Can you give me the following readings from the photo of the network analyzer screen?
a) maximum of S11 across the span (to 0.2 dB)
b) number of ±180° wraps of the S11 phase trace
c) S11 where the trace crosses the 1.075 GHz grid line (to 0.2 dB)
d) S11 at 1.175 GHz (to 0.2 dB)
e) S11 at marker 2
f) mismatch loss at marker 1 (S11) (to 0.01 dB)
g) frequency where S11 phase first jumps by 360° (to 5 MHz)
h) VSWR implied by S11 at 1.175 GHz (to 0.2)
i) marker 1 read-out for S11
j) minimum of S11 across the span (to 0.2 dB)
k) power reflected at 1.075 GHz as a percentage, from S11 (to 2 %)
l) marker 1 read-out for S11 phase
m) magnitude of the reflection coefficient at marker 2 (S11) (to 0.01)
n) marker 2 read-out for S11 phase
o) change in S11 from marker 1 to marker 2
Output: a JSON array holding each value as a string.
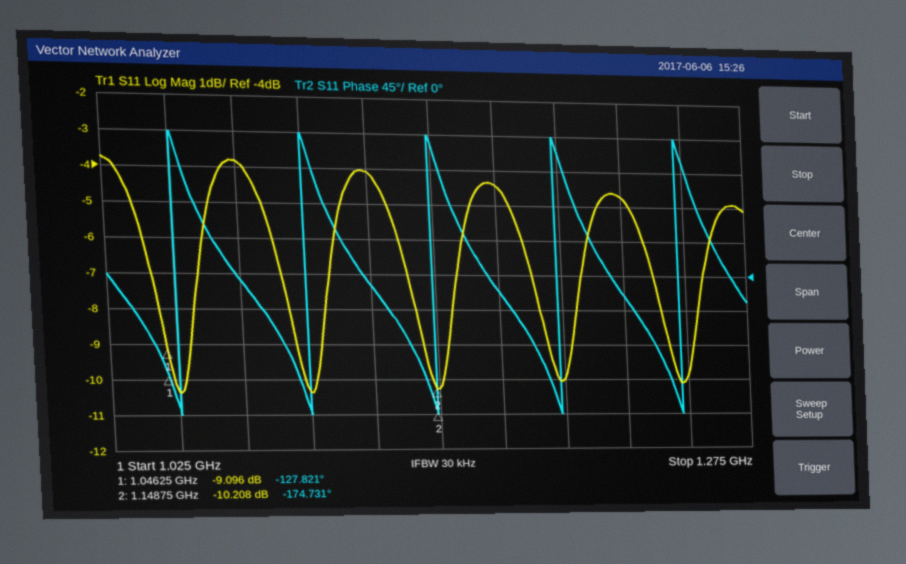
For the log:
["-3.8 dB", "5", "-3.8 dB", "-4.4 dB", "-10.208 dB", "0.57 dB", "1.050 GHz", "4.0", "-9.096 dB", "-10.4 dB", "42 %", "-127.821°", "0.31", "-174.731°", "-1.112 dB"]
